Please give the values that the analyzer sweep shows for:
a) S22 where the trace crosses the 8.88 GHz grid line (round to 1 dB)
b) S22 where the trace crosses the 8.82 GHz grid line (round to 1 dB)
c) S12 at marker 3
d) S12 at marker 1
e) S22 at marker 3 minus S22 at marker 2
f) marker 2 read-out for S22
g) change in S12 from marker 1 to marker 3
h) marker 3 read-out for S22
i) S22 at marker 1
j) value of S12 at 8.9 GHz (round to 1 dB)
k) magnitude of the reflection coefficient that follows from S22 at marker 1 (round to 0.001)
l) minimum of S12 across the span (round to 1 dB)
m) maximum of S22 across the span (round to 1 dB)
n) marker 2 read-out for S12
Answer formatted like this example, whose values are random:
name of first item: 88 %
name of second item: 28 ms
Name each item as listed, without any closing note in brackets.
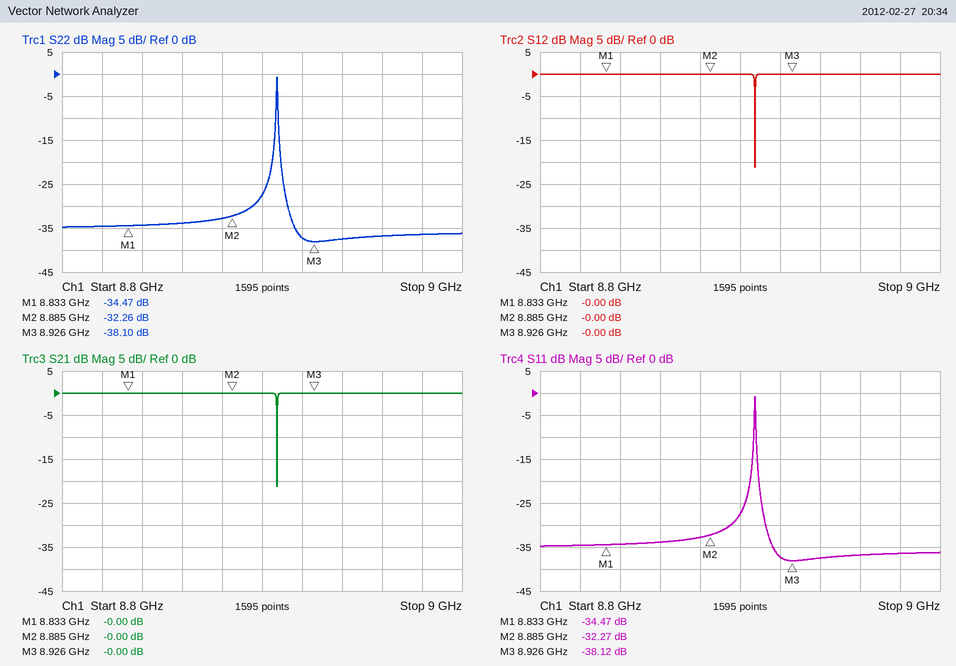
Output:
S22 where the trace crosses the 8.88 GHz grid line: -33 dB
S22 where the trace crosses the 8.82 GHz grid line: -35 dB
S12 at marker 3: -0.00 dB
S12 at marker 1: -0.00 dB
S22 at marker 3 minus S22 at marker 2: -5.84 dB
marker 2 read-out for S22: -32.26 dB
change in S12 from marker 1 to marker 3: 0.00 dB
marker 3 read-out for S22: -38.10 dB
S22 at marker 1: -34.47 dB
value of S12 at 8.9 GHz: 0 dB
magnitude of the reflection coefficient that follows from S22 at marker 1: 0.019
minimum of S12 across the span: -21 dB
maximum of S22 across the span: -1 dB
marker 2 read-out for S12: -0.00 dB
